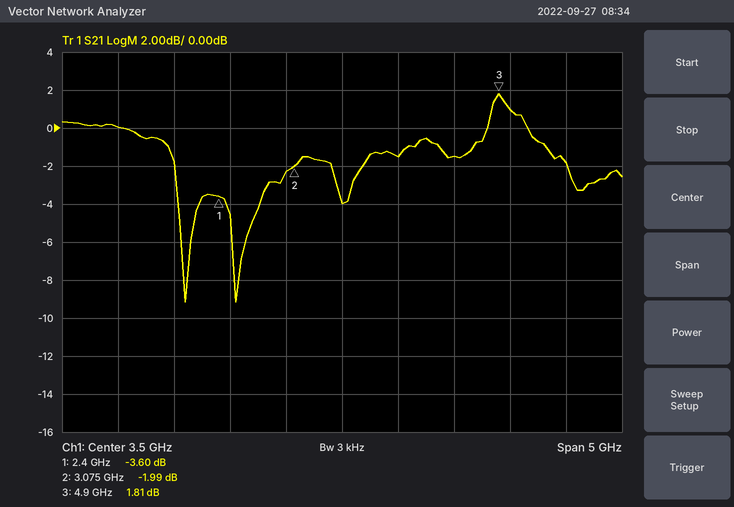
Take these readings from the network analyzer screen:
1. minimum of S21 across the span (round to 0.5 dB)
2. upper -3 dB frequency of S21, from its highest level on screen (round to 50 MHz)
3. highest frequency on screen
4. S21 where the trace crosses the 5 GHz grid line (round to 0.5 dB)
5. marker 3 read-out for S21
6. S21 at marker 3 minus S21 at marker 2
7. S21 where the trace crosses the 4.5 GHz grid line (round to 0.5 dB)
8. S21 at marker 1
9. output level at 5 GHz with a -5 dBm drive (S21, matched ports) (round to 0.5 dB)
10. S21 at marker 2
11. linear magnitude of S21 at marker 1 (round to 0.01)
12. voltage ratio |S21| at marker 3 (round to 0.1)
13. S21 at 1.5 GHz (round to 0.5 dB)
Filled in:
-9.0 dB
5.35 GHz
6 GHz
1.0 dB
1.81 dB
3.80 dB
-1.5 dB
-3.60 dB
-4.0 dBm
-1.99 dB
0.66
1.2
0.0 dB
